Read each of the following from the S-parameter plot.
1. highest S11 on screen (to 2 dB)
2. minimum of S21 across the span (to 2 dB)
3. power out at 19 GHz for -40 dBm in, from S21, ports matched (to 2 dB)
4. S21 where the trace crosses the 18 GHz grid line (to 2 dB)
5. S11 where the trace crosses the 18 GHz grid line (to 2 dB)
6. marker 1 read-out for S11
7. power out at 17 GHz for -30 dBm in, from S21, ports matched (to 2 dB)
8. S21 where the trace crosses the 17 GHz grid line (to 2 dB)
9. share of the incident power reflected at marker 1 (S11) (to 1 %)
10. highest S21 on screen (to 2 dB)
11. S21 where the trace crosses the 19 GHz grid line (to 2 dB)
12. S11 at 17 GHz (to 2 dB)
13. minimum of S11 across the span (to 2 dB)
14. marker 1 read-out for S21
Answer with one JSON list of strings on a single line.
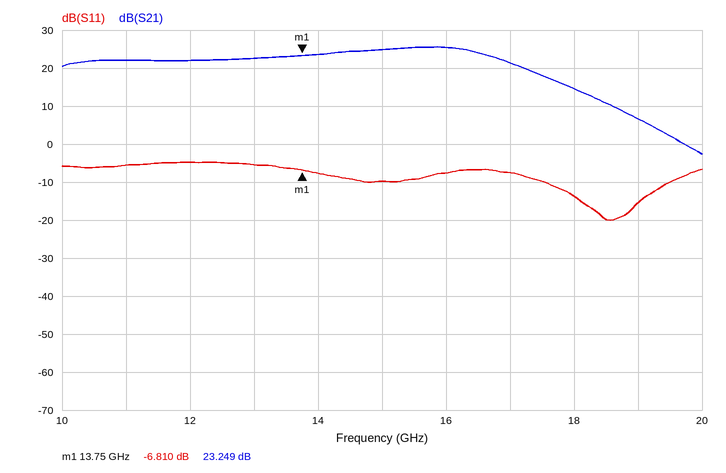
["-4 dB", "-2 dB", "-34 dBm", "14 dB", "-14 dB", "-6.810 dB", "-8 dBm", "22 dB", "21 %", "26 dB", "6 dB", "-8 dB", "-20 dB", "23.249 dB"]
